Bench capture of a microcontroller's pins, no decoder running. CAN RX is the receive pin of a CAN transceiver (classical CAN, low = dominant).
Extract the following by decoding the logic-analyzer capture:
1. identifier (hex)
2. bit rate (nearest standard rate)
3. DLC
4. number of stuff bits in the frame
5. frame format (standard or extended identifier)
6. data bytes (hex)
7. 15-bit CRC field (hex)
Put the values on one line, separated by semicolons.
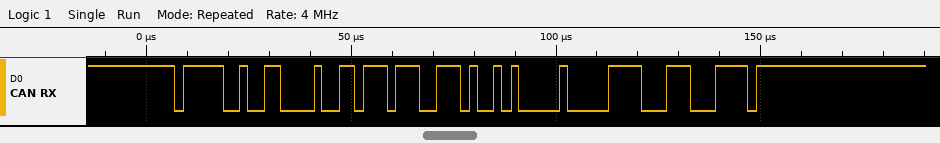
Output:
0x7D3; 500 kbit/s; 4; 3; standard; DD CE 94 00; 0x71C7
